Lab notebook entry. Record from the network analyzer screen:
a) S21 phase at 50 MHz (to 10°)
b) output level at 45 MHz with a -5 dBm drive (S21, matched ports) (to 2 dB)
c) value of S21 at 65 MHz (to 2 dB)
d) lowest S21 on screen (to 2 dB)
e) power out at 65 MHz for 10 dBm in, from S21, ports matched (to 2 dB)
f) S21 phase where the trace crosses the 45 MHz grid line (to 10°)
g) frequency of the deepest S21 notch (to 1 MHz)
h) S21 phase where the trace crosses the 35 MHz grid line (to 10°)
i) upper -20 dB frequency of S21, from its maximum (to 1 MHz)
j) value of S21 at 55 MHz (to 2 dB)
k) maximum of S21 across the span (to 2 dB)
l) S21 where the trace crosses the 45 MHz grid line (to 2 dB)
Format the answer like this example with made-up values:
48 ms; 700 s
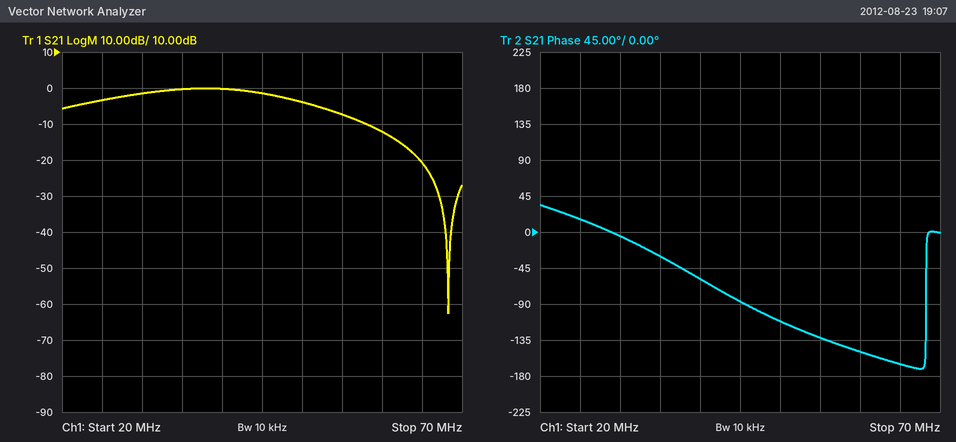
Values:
-110°; -6 dBm; -20 dB; -62 dB; -10 dBm; -90°; 68 MHz; -30°; 65 MHz; -8 dB; 0 dB; -2 dB
